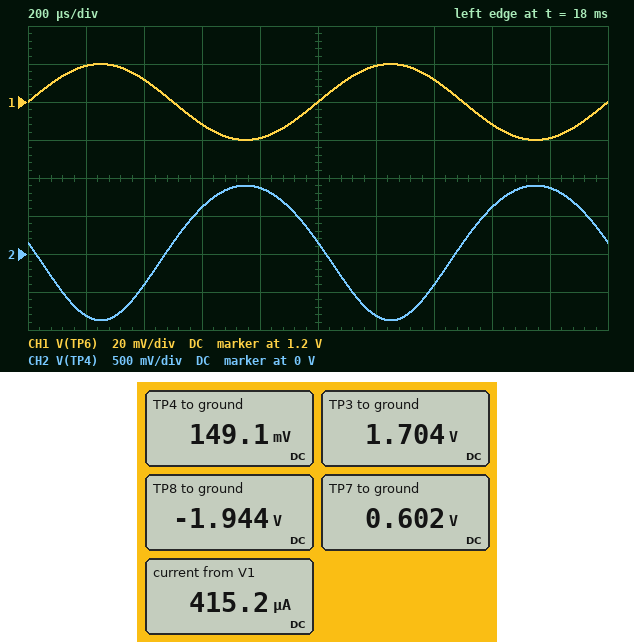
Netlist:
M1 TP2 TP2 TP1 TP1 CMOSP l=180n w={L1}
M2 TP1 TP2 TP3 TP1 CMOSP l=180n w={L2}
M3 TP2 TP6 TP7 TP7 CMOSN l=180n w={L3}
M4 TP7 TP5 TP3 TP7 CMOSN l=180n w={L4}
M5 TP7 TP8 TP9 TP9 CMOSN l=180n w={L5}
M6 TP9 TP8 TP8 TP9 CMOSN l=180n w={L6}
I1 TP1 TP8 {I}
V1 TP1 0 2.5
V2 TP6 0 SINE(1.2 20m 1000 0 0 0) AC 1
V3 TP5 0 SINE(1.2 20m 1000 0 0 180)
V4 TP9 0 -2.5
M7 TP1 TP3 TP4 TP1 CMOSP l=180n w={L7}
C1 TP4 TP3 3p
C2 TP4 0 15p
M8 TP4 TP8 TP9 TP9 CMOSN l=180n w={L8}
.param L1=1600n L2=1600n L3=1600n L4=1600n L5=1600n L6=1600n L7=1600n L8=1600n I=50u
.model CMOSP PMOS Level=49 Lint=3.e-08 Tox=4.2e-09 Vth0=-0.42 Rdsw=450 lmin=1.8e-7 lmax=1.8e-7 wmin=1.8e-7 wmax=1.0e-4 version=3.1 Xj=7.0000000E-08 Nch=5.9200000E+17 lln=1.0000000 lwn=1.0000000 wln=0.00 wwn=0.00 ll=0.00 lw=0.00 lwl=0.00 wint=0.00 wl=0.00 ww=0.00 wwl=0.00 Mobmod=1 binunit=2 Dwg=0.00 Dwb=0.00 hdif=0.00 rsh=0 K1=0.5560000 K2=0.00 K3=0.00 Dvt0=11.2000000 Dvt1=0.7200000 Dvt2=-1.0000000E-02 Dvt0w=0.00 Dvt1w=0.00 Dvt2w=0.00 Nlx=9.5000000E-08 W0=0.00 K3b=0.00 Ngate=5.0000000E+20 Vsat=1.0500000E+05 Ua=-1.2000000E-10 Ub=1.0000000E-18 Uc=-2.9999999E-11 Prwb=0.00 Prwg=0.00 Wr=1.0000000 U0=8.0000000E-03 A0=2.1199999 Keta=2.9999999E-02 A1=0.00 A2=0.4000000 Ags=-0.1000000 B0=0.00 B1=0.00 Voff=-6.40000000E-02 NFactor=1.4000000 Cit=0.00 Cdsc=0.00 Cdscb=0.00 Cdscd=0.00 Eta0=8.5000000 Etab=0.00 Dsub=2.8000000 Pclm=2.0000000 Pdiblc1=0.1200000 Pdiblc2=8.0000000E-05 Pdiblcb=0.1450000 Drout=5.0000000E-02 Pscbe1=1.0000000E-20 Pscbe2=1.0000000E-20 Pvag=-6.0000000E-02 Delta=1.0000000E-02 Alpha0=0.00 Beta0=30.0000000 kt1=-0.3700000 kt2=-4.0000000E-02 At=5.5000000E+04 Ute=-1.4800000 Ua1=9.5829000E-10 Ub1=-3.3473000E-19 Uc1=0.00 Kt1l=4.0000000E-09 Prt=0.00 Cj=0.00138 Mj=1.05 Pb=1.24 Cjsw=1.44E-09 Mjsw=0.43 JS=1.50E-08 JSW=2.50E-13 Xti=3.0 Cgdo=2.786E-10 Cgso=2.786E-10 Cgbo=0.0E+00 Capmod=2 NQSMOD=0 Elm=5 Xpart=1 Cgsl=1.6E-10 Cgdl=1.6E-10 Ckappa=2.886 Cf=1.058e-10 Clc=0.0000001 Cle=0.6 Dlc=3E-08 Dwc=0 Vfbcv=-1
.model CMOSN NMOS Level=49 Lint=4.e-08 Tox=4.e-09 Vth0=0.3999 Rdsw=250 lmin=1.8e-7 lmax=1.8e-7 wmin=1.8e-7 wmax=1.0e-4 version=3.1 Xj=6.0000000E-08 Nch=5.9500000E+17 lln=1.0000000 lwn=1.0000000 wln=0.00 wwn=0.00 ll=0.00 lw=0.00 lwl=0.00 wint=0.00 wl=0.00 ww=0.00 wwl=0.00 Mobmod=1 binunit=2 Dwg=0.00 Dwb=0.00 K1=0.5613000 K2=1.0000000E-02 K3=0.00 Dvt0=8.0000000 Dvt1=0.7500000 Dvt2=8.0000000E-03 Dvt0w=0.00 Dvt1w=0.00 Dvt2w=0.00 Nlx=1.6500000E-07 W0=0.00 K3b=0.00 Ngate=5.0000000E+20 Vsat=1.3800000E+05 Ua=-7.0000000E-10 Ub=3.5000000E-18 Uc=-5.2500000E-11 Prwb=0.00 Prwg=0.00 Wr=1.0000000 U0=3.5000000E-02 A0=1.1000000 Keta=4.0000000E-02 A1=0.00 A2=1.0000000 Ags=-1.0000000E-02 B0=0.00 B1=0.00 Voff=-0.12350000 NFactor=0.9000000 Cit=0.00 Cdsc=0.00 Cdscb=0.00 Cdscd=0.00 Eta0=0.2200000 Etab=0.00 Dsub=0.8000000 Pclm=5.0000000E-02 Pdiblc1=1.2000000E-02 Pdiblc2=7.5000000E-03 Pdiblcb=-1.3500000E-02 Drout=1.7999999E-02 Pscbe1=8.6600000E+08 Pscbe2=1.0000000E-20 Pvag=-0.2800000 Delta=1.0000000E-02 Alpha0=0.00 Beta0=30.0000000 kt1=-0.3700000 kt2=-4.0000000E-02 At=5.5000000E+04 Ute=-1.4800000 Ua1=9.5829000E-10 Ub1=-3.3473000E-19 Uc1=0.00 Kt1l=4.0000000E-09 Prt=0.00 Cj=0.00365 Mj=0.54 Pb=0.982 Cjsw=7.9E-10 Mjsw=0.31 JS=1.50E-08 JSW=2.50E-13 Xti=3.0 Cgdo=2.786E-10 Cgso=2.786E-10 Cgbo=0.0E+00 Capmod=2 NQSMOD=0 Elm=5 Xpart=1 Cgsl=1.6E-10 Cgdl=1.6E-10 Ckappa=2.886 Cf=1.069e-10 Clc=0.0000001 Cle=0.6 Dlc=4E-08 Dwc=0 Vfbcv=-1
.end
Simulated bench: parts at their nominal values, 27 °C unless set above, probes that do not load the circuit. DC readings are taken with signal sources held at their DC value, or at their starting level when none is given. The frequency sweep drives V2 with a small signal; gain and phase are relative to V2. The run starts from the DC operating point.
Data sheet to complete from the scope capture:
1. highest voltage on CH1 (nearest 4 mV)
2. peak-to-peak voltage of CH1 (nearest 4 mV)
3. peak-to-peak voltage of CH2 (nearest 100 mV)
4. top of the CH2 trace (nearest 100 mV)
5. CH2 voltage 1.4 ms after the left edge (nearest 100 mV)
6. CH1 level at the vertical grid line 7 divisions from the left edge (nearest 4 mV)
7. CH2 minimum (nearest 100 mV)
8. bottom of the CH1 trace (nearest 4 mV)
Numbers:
1.220 V
40 mV
1.8 V
900 mV
-400 mV
1.212 V
-900 mV
1.180 V
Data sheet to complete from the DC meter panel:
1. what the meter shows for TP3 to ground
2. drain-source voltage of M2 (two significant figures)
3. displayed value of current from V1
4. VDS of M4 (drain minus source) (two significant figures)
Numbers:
1.704 V
800 mV
415.2 µA
-1.1 V
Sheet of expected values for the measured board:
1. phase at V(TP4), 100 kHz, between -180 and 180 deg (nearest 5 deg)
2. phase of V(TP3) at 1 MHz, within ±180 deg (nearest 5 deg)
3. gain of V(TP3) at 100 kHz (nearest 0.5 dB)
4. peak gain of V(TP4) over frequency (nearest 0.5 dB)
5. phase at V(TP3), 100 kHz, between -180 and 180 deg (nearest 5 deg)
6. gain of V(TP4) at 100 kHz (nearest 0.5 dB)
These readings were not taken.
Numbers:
170 deg
-20 deg
15.0 dB
26.5 dB
-5 deg
26.5 dB
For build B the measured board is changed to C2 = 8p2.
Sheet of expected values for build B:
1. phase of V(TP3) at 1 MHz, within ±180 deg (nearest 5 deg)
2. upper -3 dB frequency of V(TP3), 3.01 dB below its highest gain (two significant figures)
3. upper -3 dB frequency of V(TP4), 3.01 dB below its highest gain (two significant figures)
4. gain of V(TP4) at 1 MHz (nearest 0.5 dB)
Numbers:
-30 deg
820 kHz
660 kHz
21.5 dB
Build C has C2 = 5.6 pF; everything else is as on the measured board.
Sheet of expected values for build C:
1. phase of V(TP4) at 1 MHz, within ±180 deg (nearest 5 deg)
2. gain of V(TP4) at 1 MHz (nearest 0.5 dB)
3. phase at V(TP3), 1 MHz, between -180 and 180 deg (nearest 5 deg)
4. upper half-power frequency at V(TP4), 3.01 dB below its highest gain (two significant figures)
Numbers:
120 deg
22.0 dB
-30 deg
730 kHz
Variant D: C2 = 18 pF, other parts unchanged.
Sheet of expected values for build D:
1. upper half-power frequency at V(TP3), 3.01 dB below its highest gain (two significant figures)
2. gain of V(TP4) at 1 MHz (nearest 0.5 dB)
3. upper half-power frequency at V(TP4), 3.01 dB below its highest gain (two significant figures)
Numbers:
860 kHz
19.5 dB
500 kHz
